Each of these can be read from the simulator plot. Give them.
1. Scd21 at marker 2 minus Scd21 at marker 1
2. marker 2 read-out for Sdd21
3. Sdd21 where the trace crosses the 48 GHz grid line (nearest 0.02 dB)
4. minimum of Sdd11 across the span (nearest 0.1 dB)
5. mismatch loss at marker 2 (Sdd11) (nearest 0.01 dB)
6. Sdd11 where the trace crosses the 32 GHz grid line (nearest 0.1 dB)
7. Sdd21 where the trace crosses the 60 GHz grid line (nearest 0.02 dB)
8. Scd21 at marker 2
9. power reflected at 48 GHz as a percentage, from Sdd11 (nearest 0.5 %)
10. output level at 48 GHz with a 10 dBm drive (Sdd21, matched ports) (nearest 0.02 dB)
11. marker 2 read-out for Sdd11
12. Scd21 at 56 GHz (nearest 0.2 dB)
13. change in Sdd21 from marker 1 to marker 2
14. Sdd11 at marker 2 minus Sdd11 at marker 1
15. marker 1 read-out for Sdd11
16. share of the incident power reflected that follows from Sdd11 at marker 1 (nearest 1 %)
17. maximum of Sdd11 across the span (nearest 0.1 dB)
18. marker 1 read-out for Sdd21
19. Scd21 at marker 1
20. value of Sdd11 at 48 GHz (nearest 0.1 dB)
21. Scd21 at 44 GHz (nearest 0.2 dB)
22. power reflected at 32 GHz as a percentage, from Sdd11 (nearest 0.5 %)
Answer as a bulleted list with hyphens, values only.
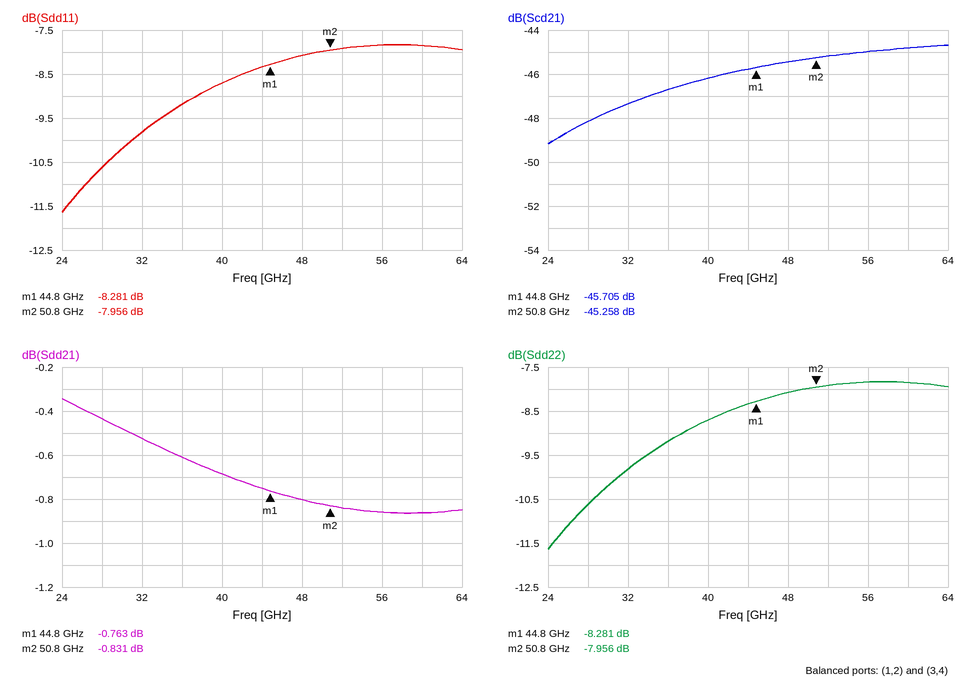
- 0.447 dB
- -0.831 dB
- -0.80 dB
- -11.6 dB
- 0.76 dB
- -9.8 dB
- -0.86 dB
- -45.258 dB
- 15.5 %
- 9.20 dBm
- -7.956 dB
- -45.0 dB
- -0.068 dB
- 0.325 dB
- -8.281 dB
- 15 %
- -7.8 dB
- -0.763 dB
- -45.705 dB
- -8.1 dB
- -45.8 dB
- 10.5 %
